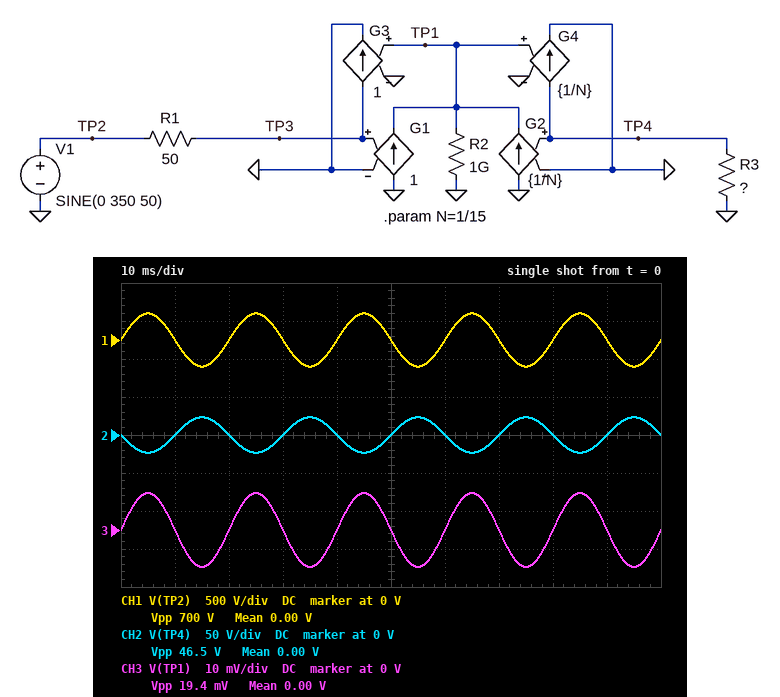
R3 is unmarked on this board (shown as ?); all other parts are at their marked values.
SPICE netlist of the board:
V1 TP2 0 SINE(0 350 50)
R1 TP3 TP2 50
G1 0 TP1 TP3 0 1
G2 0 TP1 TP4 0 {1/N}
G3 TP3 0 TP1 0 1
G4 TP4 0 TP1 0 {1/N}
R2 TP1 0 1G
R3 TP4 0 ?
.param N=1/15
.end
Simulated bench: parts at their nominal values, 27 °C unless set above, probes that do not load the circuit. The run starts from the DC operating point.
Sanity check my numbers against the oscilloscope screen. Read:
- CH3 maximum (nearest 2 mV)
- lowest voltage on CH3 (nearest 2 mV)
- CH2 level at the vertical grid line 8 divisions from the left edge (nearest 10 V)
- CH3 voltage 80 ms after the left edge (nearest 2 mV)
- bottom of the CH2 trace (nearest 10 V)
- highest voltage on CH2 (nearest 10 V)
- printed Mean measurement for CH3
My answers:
10 mV
-10 mV
0 V
0 V
-20 V
20 V
0.00 V
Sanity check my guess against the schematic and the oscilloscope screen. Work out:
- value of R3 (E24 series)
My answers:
160 Ω
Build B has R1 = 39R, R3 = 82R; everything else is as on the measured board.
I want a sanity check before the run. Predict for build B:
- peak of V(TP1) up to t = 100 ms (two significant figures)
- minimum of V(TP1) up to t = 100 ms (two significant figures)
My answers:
19 mV
-19 mV
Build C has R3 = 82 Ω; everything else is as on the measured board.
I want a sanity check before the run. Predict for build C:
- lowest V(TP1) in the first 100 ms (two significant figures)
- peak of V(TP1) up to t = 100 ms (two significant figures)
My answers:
-19 mV
19 mV
